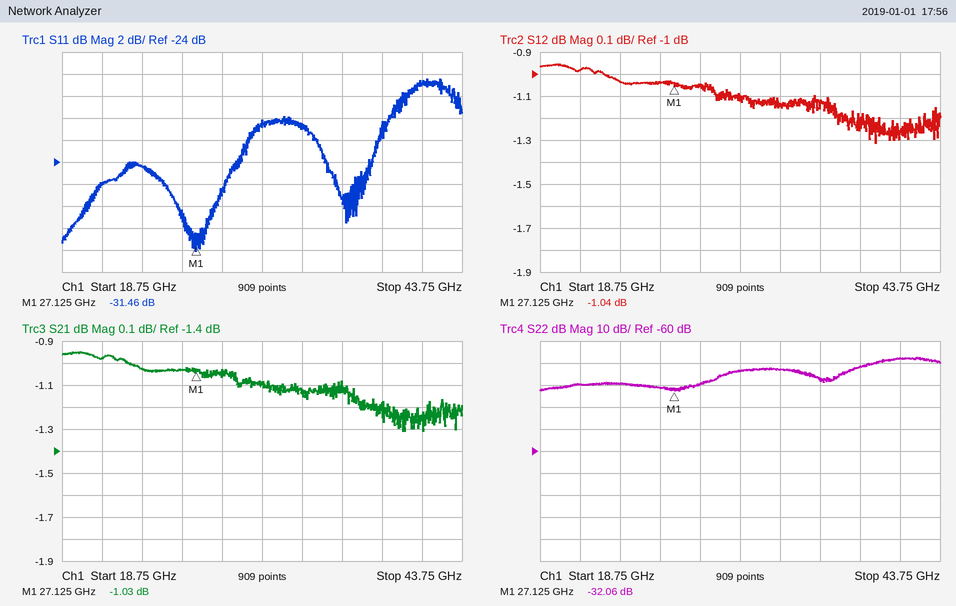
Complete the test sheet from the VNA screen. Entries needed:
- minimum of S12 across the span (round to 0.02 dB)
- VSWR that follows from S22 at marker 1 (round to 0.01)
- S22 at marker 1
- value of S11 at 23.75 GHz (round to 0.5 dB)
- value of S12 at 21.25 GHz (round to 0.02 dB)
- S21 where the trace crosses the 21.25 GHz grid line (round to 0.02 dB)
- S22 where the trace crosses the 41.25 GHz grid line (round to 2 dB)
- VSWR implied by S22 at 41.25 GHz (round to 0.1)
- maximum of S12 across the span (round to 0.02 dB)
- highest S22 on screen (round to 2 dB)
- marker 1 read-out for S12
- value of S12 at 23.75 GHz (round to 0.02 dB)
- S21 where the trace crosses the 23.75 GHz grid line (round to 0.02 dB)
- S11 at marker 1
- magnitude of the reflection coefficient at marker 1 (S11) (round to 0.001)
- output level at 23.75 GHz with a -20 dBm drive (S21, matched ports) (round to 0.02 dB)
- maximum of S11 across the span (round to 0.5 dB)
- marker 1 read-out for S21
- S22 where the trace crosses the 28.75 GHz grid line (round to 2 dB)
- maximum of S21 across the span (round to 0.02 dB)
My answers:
-1.32 dB
1.05
-32.06 dB
-24.5 dB
-0.98 dB
-0.98 dB
-18 dB
1.3
-0.96 dB
-18 dB
-1.04 dB
-1.04 dB
-1.02 dB
-31.46 dB
0.027
-21.02 dBm
-16.5 dB
-1.03 dB
-30 dB
-0.94 dB
